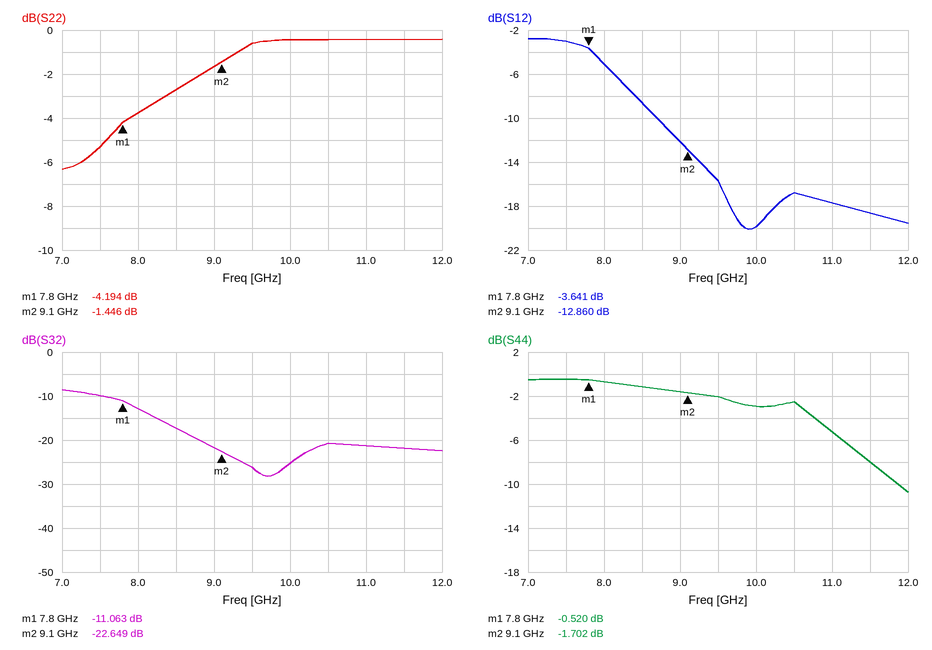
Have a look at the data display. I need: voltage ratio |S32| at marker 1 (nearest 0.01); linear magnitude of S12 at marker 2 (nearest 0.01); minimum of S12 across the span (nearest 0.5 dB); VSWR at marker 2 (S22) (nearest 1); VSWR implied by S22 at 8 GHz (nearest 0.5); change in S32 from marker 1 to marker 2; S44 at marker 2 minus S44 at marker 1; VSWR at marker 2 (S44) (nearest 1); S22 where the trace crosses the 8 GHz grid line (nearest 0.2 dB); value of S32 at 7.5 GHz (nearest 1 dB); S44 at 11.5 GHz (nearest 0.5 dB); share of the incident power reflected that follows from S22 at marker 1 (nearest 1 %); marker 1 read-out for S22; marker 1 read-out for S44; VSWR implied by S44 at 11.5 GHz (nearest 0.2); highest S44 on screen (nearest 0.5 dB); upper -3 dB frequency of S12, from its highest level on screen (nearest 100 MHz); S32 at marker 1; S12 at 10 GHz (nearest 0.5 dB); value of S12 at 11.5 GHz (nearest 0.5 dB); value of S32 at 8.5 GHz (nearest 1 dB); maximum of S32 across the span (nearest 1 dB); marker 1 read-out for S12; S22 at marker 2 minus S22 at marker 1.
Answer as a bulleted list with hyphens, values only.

- 0.28
- 0.23
- -20.0 dB
- 12
- 4.5
- -11.586 dB
- -1.182 dB
- 10
- -3.8 dB
- -10 dB
- -8.0 dB
- 38 %
- -4.194 dB
- -0.520 dB
- 2.4
- -0.5 dB
- 8.1 GHz
- -11.063 dB
- -20.0 dB
- -18.5 dB
- -17 dB
- -9 dB
- -3.641 dB
- 2.748 dB
